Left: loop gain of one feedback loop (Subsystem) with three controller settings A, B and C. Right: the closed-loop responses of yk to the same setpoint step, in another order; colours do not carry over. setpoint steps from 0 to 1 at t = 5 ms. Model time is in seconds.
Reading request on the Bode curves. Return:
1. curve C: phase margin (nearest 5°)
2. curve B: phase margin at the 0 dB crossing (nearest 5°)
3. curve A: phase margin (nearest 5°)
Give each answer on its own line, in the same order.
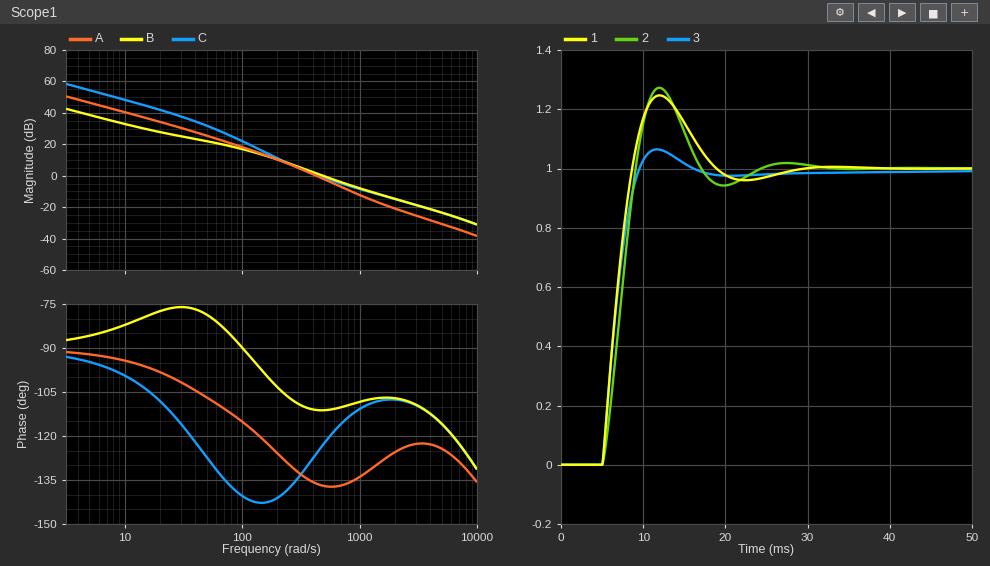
55°
70°
45°
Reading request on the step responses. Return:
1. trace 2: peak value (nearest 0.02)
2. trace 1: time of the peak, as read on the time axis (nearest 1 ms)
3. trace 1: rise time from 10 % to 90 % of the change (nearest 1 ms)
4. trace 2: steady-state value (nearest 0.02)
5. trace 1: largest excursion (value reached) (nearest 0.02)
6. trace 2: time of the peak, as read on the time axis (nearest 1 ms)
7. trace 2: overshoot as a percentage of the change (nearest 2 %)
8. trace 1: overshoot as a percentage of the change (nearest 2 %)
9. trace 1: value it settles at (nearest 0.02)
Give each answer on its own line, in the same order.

1.28
12 ms
3 ms
1.00
1.24
12 ms
28 %
24 %
1.00
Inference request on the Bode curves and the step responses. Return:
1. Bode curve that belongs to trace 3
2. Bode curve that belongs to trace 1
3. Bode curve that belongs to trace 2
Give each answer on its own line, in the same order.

B
C
A
